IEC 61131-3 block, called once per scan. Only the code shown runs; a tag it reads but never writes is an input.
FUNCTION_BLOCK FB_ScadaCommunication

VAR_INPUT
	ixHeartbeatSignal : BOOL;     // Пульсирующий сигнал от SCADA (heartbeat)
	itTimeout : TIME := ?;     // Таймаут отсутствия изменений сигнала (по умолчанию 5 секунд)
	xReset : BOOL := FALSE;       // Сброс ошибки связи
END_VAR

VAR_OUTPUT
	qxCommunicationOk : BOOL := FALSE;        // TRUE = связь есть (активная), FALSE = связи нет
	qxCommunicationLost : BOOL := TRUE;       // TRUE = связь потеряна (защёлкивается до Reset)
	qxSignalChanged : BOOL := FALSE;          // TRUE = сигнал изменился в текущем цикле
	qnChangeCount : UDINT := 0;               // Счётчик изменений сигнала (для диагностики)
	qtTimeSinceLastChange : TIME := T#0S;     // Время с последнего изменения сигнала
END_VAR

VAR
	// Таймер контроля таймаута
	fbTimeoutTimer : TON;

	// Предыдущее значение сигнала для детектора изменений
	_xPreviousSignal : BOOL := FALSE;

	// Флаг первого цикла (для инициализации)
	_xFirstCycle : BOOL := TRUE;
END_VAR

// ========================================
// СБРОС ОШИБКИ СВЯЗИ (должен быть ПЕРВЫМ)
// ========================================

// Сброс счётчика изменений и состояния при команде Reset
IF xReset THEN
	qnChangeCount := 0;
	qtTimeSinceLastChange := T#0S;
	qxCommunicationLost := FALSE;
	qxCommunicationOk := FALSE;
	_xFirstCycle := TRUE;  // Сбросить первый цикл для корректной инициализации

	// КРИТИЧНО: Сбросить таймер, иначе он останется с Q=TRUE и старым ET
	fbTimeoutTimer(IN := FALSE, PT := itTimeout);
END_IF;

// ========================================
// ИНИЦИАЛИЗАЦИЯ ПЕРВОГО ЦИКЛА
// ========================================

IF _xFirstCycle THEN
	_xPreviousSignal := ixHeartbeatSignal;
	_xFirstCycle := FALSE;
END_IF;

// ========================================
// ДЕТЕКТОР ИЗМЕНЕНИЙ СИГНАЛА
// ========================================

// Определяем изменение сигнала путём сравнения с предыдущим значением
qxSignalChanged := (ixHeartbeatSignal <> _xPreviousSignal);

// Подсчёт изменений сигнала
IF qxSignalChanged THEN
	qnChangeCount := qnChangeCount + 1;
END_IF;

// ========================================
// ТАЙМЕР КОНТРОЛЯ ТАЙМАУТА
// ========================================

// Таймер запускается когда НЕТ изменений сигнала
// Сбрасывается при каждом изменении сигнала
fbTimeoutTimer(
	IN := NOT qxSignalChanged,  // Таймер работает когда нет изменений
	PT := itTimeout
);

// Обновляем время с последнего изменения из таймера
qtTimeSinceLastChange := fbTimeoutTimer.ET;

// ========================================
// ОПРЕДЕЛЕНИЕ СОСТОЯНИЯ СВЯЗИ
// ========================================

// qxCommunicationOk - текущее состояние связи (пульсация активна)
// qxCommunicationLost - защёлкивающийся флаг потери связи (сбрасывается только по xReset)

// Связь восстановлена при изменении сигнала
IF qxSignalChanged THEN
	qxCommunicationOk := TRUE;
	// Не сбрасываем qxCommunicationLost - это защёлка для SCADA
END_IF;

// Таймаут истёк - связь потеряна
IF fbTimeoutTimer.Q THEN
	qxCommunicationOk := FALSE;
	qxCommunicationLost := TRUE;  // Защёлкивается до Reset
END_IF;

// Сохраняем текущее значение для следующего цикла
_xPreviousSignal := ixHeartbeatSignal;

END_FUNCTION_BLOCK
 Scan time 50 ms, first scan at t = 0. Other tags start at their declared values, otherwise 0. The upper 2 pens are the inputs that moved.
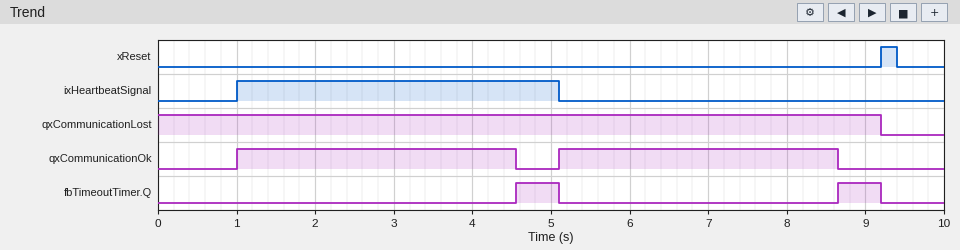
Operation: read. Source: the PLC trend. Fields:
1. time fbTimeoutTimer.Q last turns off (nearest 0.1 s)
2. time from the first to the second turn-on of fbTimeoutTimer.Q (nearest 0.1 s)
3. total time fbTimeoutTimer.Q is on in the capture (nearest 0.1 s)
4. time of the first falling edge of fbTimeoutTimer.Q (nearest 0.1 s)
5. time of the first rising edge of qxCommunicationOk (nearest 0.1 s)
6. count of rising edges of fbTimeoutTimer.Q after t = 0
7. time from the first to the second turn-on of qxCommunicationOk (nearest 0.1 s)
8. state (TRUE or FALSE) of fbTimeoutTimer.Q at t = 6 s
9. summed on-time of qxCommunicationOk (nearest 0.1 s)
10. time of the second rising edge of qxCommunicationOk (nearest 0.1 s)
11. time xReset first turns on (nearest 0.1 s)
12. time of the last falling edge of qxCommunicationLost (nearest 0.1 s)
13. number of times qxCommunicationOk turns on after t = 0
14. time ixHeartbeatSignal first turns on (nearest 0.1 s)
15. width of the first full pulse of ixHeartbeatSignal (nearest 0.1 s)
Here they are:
9.2 s
4.1 s
1.1 s
5.1 s
1.0 s
2
4.1 s
FALSE
7.1 s
5.1 s
9.2 s
9.2 s
2
1.0 s
4.1 s
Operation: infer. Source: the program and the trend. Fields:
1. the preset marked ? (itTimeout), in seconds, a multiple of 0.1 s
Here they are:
3.5 s
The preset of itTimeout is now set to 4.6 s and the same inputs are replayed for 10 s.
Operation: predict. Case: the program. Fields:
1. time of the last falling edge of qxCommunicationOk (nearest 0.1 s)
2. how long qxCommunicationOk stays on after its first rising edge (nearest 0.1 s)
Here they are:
9.2 s
8.2 s
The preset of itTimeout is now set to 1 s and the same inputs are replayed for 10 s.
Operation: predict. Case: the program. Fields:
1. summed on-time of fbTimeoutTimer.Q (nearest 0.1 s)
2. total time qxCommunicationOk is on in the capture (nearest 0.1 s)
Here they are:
6.1 s
2.1 s
